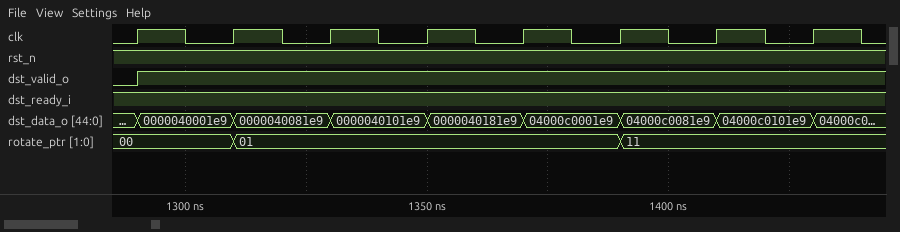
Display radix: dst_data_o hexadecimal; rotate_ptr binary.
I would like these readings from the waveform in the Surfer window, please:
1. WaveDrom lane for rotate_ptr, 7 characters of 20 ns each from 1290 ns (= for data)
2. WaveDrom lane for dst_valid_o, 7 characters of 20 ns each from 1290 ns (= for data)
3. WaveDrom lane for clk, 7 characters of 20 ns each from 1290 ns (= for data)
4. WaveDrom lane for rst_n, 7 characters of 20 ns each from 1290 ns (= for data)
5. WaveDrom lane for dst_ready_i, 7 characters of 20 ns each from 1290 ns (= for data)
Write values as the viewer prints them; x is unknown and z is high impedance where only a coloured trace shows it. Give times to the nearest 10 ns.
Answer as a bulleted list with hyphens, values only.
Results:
- {name: 'rotate_ptr', wave: '==...=.', data: '00 01 11'}
- {name: 'dst_valid_o', wave: '1......'}
- {name: 'clk', wave: 'p......'}
- {name: 'rst_n', wave: '1......'}
- {name: 'dst_ready_i', wave: '1......'}
